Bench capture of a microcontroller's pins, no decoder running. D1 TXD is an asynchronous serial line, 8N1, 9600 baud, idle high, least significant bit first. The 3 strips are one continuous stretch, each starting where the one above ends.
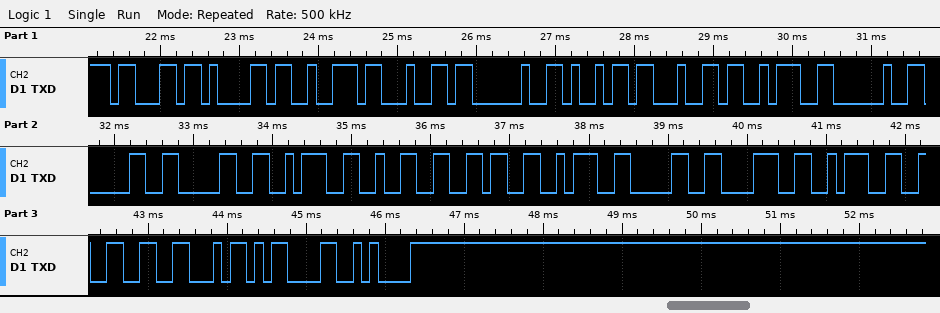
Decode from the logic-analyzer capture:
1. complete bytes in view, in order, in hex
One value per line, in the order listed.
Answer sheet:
63 61 72 64 20 69 64 3A 20 30 30 3A 32 36 3A 30 38 3A 32 46 0D 0A
